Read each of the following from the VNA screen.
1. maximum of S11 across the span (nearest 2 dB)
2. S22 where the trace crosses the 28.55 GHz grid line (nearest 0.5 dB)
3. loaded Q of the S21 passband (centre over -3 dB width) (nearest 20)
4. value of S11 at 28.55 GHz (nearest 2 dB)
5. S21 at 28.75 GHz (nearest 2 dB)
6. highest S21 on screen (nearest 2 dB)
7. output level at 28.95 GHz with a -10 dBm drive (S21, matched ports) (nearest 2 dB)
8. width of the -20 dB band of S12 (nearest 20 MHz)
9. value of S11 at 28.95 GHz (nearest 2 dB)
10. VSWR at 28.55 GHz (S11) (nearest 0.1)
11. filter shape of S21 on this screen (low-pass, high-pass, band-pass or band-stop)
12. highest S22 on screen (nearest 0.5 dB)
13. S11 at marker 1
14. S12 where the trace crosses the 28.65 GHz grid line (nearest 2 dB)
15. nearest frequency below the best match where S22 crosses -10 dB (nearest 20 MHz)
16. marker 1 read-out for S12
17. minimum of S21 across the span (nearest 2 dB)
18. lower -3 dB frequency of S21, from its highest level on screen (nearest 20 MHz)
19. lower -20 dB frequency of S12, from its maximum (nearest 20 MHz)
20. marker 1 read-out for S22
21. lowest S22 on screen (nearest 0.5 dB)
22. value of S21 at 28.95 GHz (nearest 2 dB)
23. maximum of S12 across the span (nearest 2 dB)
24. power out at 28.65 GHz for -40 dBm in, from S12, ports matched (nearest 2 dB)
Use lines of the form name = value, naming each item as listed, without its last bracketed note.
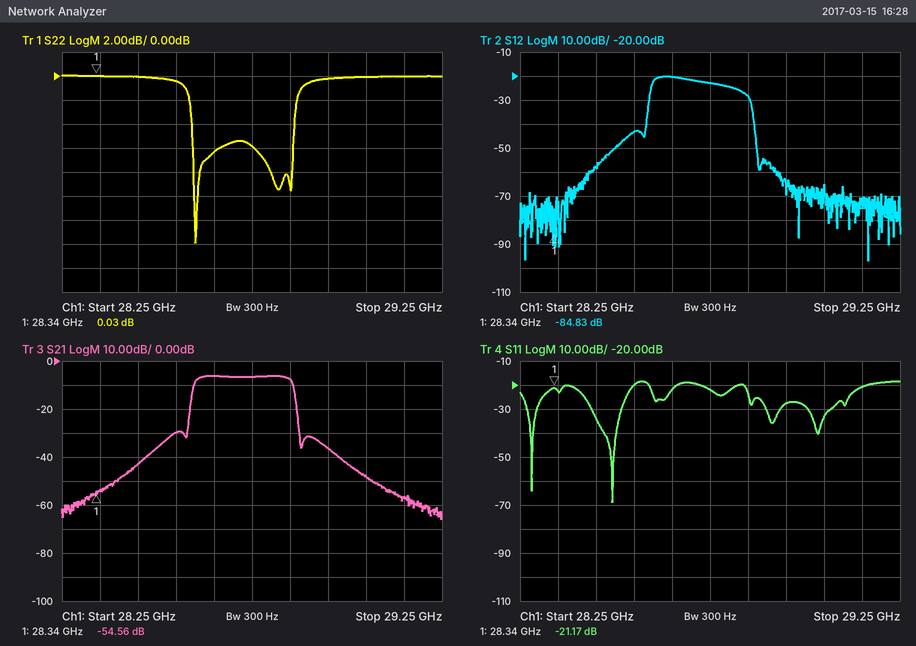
maximum of S11 across the span = -18 dB
S22 where the trace crosses the 28.55 GHz grid line = -0.5 dB
loaded Q of the S21 passband (centre over -3 dB width) = 120
value of S11 at 28.55 GHz = -20 dB
S21 at 28.75 GHz = -6 dB
highest S21 on screen = -6 dB
output level at 28.95 GHz with a -10 dBm drive (S21, matched ports) = -46 dBm
width of the -20 dB band of S12 = 280 MHz
value of S11 at 28.95 GHz = -28 dB
VSWR at 28.55 GHz (S11) = 1.2
filter shape of S21 on this screen = band-pass
highest S22 on screen = 0.0 dB
S11 at marker 1 = -21.17 dB
S12 where the trace crosses the 28.65 GHz grid line = -20 dB
nearest frequency below the best match where S22 crosses -10 dB = 28.60 GHz
marker 1 read-out for S12 = -84.83 dB
minimum of S21 across the span = -66 dB
lower -3 dB frequency of S21, from its highest level on screen = 28.60 GHz
lower -20 dB frequency of S12, from its maximum = 28.58 GHz
marker 1 read-out for S22 = 0.03 dB
lowest S22 on screen = -14.0 dB
value of S21 at 28.95 GHz = -36 dB
maximum of S12 across the span = -20 dB
power out at 28.65 GHz for -40 dBm in, from S12, ports matched = -60 dBm
